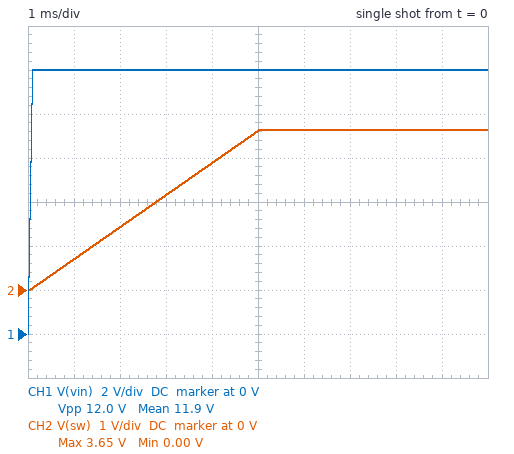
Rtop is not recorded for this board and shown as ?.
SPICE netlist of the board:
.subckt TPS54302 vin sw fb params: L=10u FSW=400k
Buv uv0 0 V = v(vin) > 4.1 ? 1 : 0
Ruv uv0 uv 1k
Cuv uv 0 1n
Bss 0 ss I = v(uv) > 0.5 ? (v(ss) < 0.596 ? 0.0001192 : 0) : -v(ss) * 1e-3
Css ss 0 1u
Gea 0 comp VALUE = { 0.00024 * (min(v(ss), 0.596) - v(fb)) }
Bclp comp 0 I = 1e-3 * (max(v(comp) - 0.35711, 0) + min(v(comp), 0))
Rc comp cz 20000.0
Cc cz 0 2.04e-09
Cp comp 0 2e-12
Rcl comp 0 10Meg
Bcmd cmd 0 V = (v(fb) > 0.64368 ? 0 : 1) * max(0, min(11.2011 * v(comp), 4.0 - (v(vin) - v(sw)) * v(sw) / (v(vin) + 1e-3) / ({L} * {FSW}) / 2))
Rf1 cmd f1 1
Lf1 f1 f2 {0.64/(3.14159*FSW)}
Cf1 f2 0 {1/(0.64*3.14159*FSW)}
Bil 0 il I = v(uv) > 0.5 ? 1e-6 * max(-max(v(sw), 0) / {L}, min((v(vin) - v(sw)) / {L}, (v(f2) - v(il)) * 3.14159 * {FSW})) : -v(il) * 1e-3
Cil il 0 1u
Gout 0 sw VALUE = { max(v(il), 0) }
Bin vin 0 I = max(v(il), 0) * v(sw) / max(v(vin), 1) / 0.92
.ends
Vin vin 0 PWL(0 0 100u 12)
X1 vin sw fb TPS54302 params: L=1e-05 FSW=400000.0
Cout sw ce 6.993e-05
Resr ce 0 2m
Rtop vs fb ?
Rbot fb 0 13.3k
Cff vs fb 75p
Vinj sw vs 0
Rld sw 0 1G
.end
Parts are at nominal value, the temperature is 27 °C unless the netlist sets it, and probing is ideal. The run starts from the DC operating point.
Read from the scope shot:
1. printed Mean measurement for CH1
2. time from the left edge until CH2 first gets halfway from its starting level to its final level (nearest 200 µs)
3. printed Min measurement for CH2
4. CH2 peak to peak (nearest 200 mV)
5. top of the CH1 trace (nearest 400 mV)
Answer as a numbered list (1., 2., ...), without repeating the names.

1. 11.9 V
2. 2.6 ms
3. 0.00 V
4. 3.6 V
5. 12.0 V
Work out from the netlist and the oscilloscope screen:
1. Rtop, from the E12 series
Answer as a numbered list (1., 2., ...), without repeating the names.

1. 68 kΩ
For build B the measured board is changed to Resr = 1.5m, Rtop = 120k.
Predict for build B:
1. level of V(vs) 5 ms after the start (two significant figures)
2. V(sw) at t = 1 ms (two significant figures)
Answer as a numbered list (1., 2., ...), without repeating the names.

1. 5.9 V
2. 1.1 V
